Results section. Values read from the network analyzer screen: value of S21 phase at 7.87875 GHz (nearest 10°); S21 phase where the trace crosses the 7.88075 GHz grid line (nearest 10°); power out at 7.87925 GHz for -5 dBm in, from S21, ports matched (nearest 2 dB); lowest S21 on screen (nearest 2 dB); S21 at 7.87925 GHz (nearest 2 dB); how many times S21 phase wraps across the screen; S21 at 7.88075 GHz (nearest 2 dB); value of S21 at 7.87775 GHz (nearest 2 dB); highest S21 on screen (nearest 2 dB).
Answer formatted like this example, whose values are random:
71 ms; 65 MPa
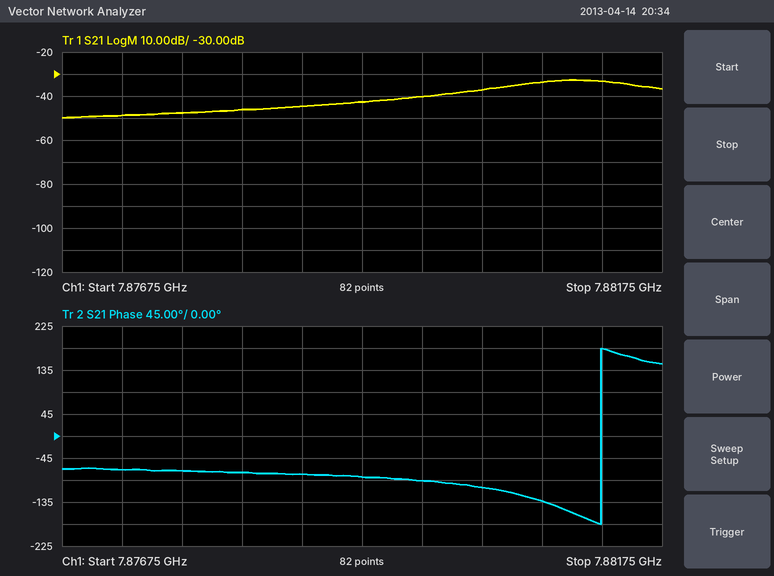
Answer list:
-80°; -130°; -48 dBm; -50 dB; -42 dB; 1; -34 dB; -48 dB; -32 dB
